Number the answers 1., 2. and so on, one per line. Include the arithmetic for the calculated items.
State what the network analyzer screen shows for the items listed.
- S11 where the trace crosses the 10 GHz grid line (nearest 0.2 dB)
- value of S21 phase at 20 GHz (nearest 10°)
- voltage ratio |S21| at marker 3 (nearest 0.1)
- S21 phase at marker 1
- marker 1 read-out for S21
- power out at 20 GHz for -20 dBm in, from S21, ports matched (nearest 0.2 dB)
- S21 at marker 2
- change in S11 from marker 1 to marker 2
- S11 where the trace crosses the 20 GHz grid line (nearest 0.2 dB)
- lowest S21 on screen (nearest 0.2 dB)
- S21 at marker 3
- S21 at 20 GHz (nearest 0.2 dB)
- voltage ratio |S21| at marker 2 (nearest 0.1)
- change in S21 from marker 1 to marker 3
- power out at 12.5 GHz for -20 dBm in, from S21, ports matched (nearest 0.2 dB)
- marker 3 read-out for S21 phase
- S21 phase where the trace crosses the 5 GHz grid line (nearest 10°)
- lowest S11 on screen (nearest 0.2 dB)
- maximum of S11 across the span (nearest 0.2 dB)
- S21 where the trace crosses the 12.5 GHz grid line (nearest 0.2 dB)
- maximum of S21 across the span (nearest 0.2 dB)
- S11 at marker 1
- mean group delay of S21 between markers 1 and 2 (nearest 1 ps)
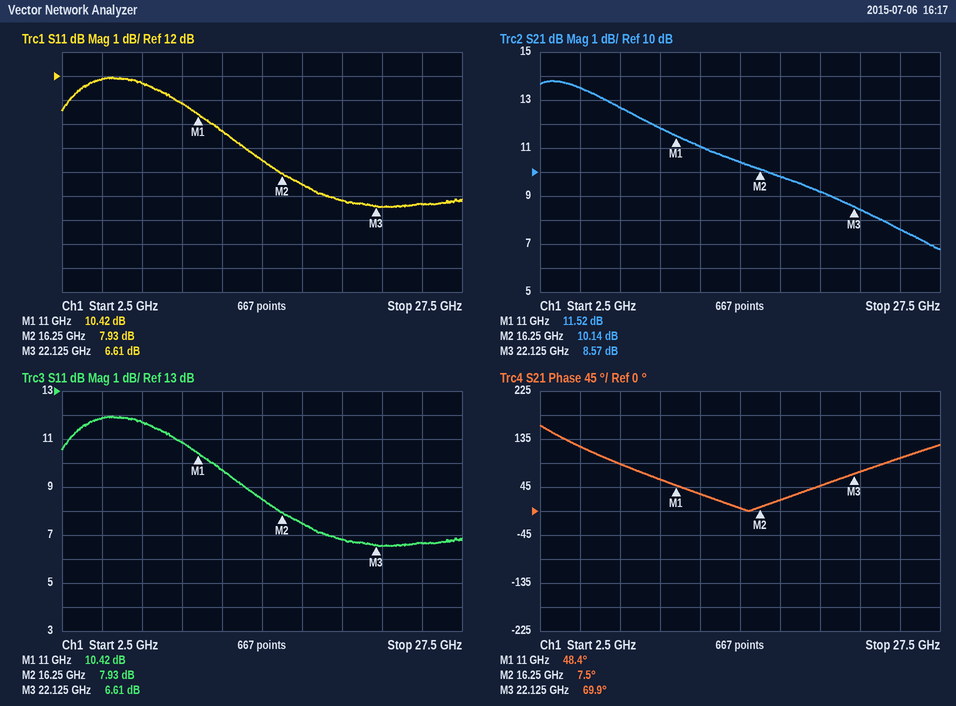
1. 10.8 dB
2. 50°
3. 10^(8.57/20) ≈ 2.7
4. 48.4°
5. 11.52 dB
6. -20 dBm + (9.2 dB) = -10.8 dBm
7. 10.14 dB
8. 7.93 − (10.42) = -2.49 dB
9. 6.8 dB
10. 6.8 dB
11. 8.57 dB
12. 9.2 dB
13. 10^(10.14/20) ≈ 3.2
14. 8.57 − (11.52) = -2.95 dB
15. -20 dBm + (11.0 dB) = -9.0 dBm
16. 69.9°
17. 120°
18. 6.6 dB
19. 12.0 dB
20. 11.0 dB
21. 13.8 dB
22. 10.42 dB
23. −(7.5° − (48.4°))/(360° × 5.25 GHz) ≈ 22 ps
